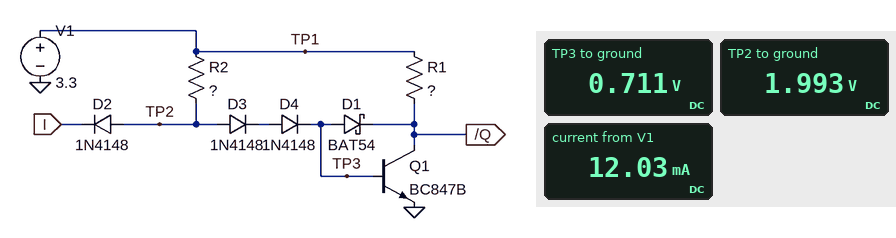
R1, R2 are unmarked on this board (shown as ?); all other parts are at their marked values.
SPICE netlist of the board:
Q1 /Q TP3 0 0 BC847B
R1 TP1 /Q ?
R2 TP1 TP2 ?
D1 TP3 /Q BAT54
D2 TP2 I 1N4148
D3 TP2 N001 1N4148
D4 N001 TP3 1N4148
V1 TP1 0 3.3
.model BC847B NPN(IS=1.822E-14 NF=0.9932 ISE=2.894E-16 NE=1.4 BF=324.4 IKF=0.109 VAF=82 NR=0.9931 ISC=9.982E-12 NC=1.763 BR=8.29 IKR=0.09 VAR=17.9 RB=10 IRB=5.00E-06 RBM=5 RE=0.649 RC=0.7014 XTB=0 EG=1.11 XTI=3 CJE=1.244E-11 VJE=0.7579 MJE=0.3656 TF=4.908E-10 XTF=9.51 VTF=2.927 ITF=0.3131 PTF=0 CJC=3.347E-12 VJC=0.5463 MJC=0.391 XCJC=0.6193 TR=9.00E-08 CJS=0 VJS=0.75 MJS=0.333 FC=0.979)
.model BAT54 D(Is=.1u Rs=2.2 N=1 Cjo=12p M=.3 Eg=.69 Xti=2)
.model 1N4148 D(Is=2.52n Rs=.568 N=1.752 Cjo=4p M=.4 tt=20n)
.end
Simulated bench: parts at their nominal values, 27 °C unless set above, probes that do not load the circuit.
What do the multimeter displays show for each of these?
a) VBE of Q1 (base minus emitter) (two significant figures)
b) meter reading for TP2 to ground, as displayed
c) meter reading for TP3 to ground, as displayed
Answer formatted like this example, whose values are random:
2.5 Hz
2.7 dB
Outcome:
710 mV
1.993 V
0.711 V
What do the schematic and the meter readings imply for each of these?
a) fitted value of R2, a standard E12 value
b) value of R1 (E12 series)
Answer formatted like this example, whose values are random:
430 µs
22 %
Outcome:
390 Ω
330 Ω
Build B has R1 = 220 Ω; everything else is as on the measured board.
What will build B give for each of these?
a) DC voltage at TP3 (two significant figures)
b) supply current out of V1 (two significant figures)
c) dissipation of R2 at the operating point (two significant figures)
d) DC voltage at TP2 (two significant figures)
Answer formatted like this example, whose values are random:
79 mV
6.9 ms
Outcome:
720 mV
16 mA
4.3 mW
2.0 V
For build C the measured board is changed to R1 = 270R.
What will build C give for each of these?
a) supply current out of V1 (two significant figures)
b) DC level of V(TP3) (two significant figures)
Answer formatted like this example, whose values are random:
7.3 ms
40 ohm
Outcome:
14 mA
720 mV
